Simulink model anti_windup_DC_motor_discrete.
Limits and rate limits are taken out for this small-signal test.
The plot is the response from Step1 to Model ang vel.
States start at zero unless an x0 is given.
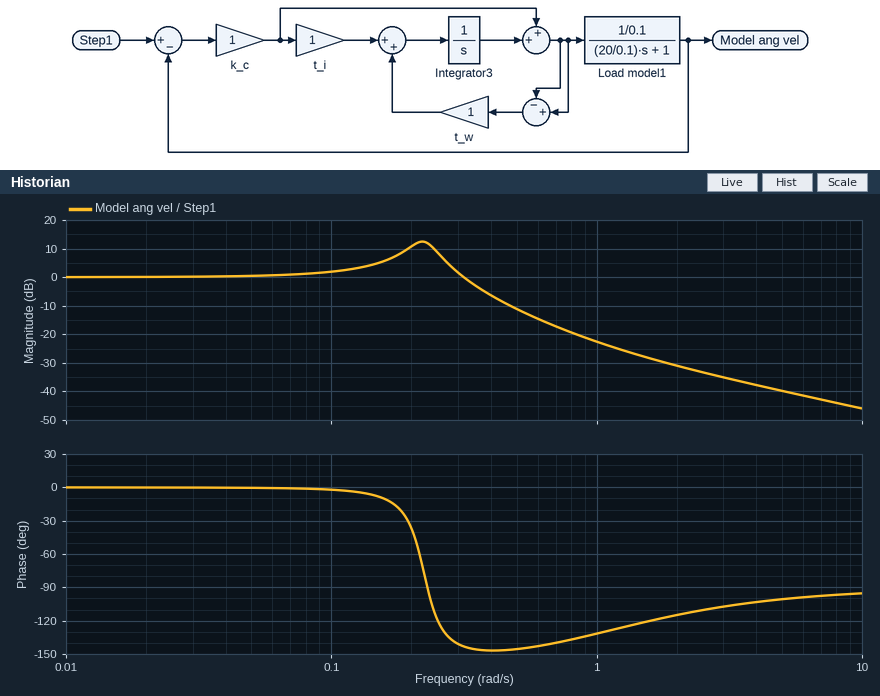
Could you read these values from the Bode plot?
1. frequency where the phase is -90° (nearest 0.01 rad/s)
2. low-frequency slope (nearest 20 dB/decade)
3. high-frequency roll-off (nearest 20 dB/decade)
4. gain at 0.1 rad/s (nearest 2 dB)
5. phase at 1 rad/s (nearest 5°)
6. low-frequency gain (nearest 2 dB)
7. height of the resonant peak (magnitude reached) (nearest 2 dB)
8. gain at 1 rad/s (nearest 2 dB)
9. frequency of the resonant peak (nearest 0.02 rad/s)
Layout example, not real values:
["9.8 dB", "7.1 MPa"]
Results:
["0.23 rad/s", "0 dB/decade", "-20 dB/decade", "2 dB", "-130°", "0 dB", "12 dB", "-22 dB", "0.22 rad/s"]
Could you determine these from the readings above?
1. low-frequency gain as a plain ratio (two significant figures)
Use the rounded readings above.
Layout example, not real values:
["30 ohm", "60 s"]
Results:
["1.0"]
